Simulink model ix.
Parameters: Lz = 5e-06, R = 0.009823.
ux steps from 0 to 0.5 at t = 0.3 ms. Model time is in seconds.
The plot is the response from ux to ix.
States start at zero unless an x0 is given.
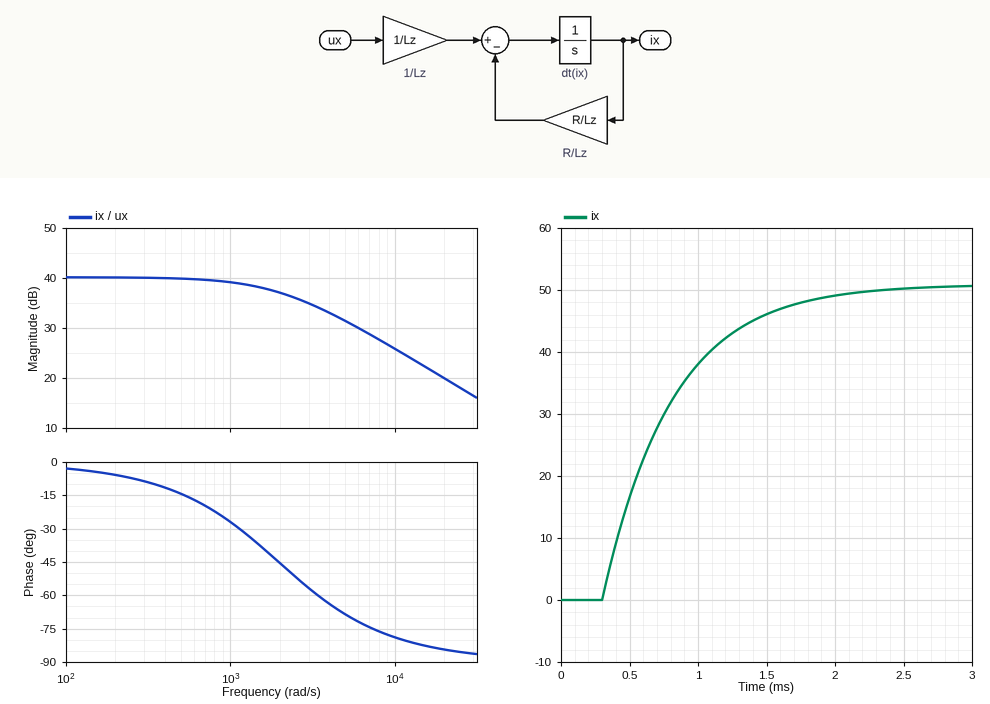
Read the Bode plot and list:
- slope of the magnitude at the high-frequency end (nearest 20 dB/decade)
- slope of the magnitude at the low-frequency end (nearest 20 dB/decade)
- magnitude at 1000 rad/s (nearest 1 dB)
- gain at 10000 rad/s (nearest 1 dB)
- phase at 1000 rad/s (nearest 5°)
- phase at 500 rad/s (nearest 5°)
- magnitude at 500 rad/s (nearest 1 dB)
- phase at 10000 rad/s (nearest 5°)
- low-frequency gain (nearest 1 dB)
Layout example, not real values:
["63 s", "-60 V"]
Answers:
["-20 dB/decade", "0 dB/decade", "39 dB", "26 dB", "-25°", "-15°", "40 dB", "-80°", "40 dB"]
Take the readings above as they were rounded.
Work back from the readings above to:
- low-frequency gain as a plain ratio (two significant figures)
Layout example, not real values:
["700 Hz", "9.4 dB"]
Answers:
["100"]
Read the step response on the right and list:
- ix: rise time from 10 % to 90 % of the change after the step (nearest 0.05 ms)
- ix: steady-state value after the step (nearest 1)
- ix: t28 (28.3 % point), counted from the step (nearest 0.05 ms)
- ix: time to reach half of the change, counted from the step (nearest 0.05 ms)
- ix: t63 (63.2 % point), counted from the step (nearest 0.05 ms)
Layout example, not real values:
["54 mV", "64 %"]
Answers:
["1.10 ms", "51", "0.15 ms", "0.35 ms", "0.50 ms"]
